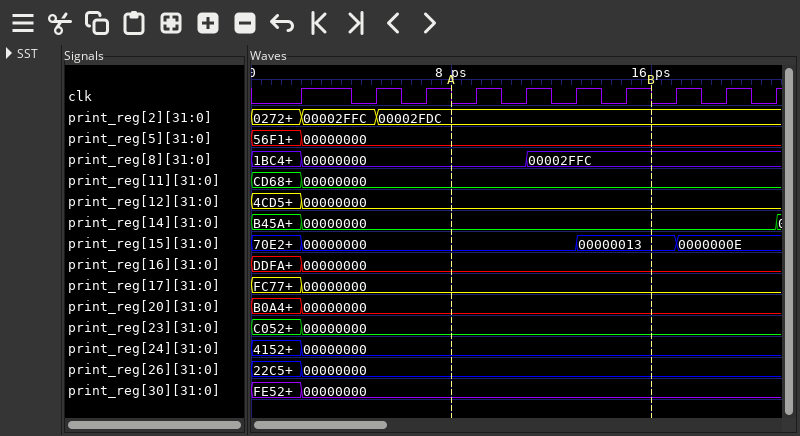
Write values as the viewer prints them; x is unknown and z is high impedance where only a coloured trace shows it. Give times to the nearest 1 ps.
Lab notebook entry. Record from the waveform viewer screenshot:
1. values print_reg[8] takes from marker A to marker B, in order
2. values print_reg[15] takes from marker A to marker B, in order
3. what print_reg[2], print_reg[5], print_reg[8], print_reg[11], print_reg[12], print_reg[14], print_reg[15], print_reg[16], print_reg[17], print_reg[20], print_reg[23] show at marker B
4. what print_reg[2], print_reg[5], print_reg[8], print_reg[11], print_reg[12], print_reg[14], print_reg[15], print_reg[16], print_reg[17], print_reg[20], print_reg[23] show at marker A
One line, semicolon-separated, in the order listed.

00000000, 00002FFC; 00000000, 00000013; print_reg[2]=00002FDC, print_reg[5]=00000000, print_reg[8]=00002FFC, print_reg[11]=00000000, print_reg[12]=00000000, print_reg[14]=00000000, print_reg[15]=00000013, print_reg[16]=00000000, print_reg[17]=00000000, print_reg[20]=00000000, print_reg[23]=00000000; print_reg[2]=00002FDC, print_reg[5]=00000000, print_reg[8]=00000000, print_reg[11]=00000000, print_reg[12]=00000000, print_reg[14]=00000000, print_reg[15]=00000000, print_reg[16]=00000000, print_reg[17]=00000000, print_reg[20]=00000000, print_reg[23]=00000000
